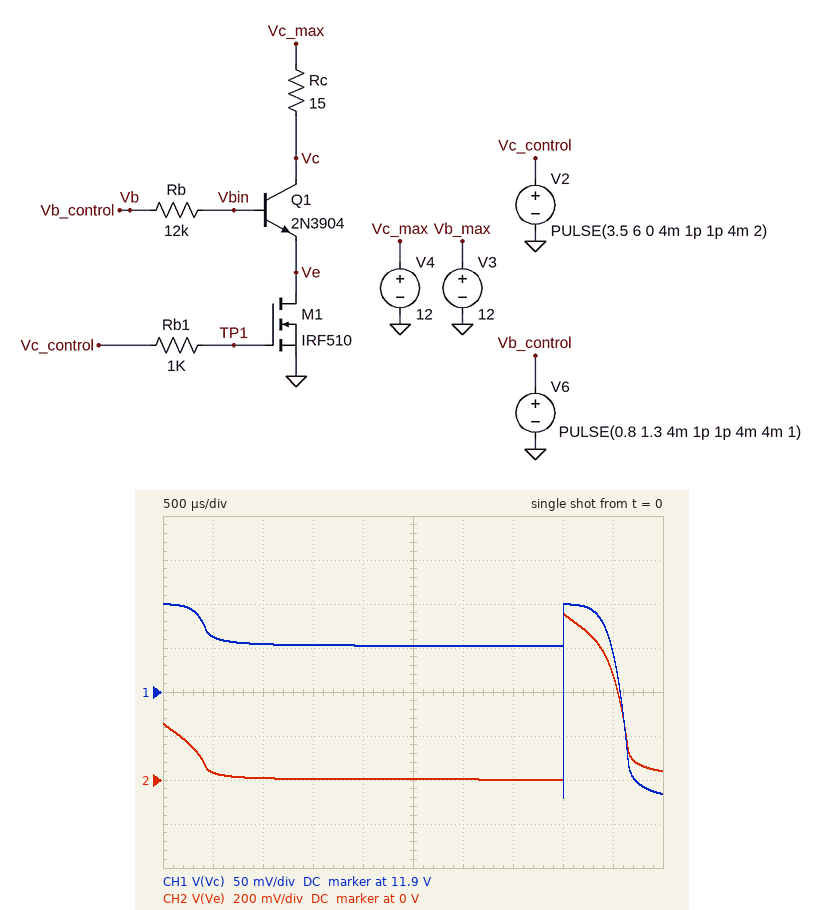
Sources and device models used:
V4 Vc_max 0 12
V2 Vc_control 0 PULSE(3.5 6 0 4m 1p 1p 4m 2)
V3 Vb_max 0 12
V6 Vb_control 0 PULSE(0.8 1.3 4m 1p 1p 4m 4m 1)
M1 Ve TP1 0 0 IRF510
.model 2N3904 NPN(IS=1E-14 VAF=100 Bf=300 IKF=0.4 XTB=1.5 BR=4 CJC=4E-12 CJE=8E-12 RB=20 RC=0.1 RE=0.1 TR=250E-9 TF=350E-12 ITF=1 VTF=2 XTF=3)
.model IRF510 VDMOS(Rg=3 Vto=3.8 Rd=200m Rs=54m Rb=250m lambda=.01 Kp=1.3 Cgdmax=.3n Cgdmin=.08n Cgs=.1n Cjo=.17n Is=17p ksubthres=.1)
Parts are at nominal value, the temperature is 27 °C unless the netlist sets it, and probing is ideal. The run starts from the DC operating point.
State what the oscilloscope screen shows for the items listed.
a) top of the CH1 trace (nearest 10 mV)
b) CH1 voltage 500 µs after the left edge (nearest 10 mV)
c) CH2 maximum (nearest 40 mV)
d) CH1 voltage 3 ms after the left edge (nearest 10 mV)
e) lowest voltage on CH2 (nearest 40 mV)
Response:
12.00 V
11.96 V
760 mV
11.95 V
0 V
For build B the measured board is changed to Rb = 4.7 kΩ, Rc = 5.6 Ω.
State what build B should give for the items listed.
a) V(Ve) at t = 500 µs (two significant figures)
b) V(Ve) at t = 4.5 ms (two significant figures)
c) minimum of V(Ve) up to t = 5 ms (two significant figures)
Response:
63 mV
560 mV
3.3 mV
